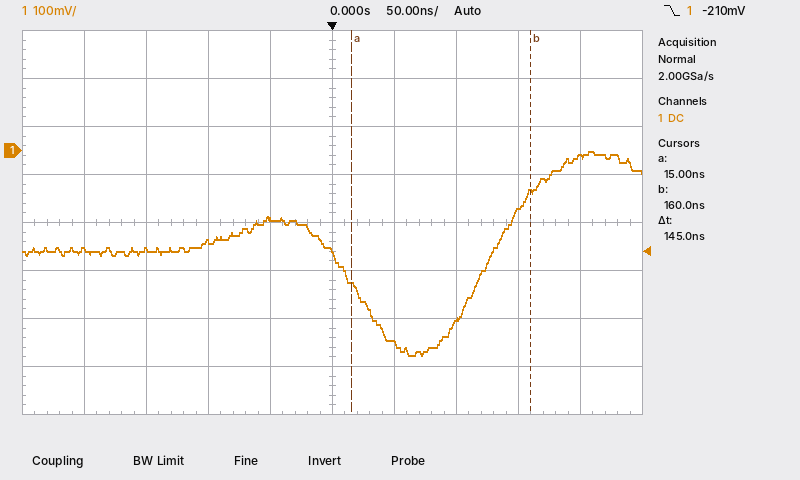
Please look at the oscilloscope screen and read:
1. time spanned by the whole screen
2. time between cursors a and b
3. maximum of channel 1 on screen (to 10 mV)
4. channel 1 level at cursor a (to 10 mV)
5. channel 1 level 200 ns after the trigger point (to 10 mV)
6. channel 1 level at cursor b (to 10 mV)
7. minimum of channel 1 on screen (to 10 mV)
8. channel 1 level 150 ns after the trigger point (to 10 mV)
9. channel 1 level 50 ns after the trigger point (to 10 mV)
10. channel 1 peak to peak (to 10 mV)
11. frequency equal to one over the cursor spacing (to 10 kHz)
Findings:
500 ns
145 ns
0 mV
-280 mV
-10 mV
-90 mV
-430 mV
-120 mV
-400 mV
430 mV
6.90 MHz
